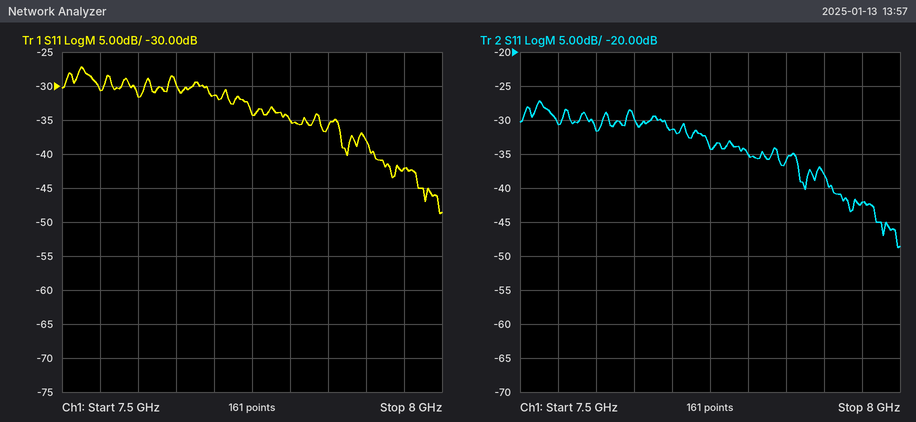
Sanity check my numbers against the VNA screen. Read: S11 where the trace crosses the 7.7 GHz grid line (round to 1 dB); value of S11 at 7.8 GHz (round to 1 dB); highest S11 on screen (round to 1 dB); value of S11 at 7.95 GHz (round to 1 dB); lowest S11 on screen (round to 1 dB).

-31 dB
-35 dB
-27 dB
-42 dB
-49 dB
